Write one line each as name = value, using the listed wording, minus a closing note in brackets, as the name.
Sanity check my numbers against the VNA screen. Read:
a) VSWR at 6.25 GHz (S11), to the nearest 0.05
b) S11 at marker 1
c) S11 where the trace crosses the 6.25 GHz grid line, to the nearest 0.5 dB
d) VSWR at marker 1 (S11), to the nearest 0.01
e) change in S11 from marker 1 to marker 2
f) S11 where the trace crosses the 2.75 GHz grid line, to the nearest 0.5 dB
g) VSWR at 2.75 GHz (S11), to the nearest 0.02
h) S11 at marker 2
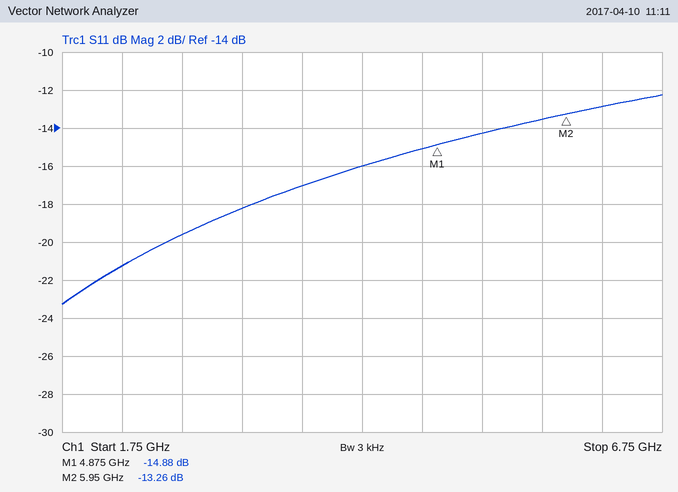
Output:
VSWR at 6.25 GHz (S11), to the nearest 0.05 = 1.60
S11 at marker 1 = -14.88 dB
S11 where the trace crosses the 6.25 GHz grid line, to the nearest 0.5 dB = -13.0 dB
VSWR at marker 1 (S11), to the nearest 0.01 = 1.44
change in S11 from marker 1 to marker 2 = 1.62 dB
S11 where the trace crosses the 2.75 GHz grid line, to the nearest 0.5 dB = -19.5 dB
VSWR at 2.75 GHz (S11), to the nearest 0.02 = 1.24
S11 at marker 2 = -13.26 dB
